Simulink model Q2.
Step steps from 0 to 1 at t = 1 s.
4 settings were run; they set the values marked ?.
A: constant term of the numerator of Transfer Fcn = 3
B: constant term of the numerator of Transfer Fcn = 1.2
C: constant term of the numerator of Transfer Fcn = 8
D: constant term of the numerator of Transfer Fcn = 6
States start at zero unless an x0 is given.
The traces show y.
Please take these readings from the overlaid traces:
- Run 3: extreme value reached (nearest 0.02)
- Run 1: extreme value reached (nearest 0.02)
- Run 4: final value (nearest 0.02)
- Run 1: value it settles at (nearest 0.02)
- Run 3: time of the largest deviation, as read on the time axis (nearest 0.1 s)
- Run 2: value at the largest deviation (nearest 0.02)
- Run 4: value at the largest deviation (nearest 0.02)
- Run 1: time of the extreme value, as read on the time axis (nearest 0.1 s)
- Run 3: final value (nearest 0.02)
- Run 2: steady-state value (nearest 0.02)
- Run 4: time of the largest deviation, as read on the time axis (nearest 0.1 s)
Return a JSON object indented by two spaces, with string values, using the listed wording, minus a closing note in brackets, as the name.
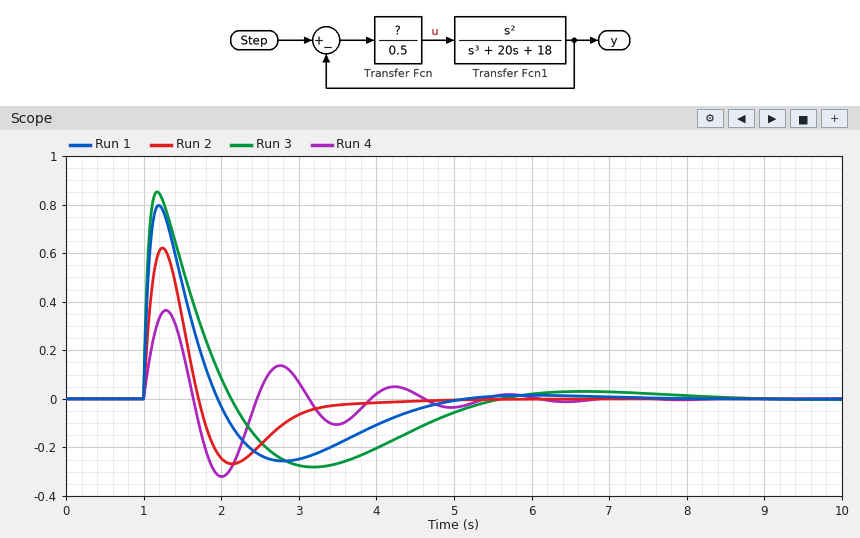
{
  "Run 3: extreme value reached": "0.86",
  "Run 1: extreme value reached": "0.80",
  "Run 4: final value": "0.00",
  "Run 1: value it settles at": "0.00",
  "Run 3: time of the largest deviation, as read on the time axis": "1.2 s",
  "Run 2: value at the largest deviation": "0.62",
  "Run 4: value at the largest deviation": "0.36",
  "Run 1: time of the extreme value, as read on the time axis": "1.2 s",
  "Run 3: final value": "0.00",
  "Run 2: steady-state value": "0.00",
  "Run 4: time of the largest deviation, as read on the time axis": "1.3 s"
}
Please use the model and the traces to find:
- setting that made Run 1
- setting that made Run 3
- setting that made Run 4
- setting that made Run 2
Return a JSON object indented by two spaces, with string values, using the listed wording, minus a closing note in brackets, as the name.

{
  "setting that made Run 1": "D",
  "setting that made Run 3": "C",
  "setting that made Run 4": "B",
  "setting that made Run 2": "A"
}
